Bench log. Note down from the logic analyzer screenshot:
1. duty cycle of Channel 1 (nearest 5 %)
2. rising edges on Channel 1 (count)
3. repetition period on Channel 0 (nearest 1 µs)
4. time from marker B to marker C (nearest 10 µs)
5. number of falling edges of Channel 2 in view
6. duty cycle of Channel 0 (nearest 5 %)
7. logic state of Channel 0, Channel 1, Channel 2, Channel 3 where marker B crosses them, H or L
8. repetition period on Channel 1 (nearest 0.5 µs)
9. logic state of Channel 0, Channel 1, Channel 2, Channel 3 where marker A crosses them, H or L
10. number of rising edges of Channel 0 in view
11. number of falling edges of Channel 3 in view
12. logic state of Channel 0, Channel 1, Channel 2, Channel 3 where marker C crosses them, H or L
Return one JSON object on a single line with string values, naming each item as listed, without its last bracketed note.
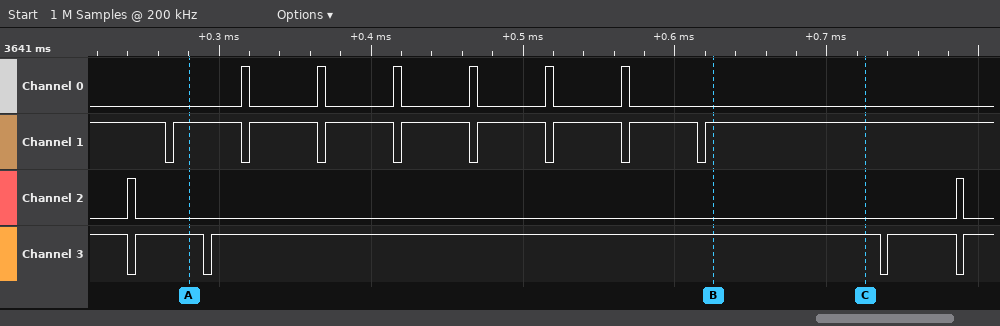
{"duty cycle of Channel 1": "90 %", "rising edges on Channel 1": "8", "repetition period on Channel 0": "50 µs", "time from marker B to marker C": "100 µs", "number of falling edges of Channel 2 in view": "2", "duty cycle of Channel 0": "10 %", "logic state of Channel 0, Channel 1, Channel 2, Channel 3 where marker B crosses them, H or L": "Channel 0=L, Channel 1=H, Channel 2=L, Channel 3=H", "repetition period on Channel 1": "50 µs", "logic state of Channel 0, Channel 1, Channel 2, Channel 3 where marker A crosses them, H or L": "Channel 0=L, Channel 1=H, Channel 2=L, Channel 3=H", "number of rising edges of Channel 0 in view": "6", "number of falling edges of Channel 3 in view": "4", "logic state of Channel 0, Channel 1, Channel 2, Channel 3 where marker C crosses them, H or L": "Channel 0=L, Channel 1=H, Channel 2=L, Channel 3=H"}
